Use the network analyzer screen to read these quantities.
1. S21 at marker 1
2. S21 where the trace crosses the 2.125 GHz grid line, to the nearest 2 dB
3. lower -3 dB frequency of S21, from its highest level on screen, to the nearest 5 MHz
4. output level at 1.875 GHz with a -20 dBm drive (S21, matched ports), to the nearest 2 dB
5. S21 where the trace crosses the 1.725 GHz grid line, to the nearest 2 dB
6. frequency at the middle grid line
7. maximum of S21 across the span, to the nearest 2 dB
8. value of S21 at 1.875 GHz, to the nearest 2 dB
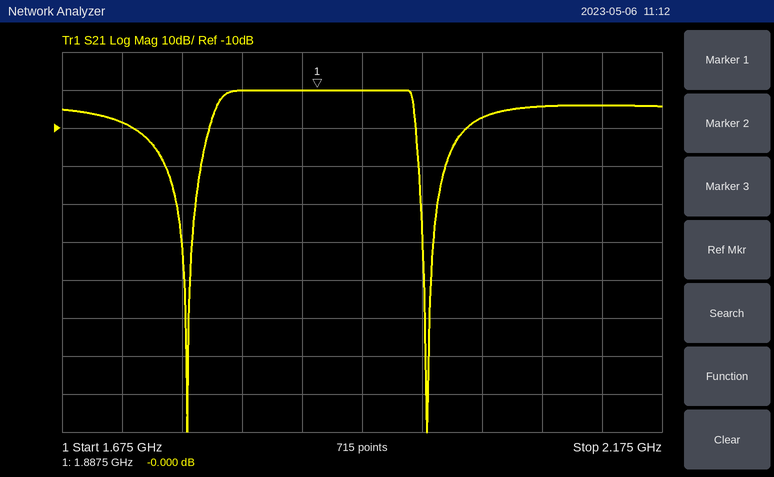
-0.000 dB
-4 dB
1.805 GHz
-20 dBm
-8 dB
1.925 GHz
0 dB
0 dB
